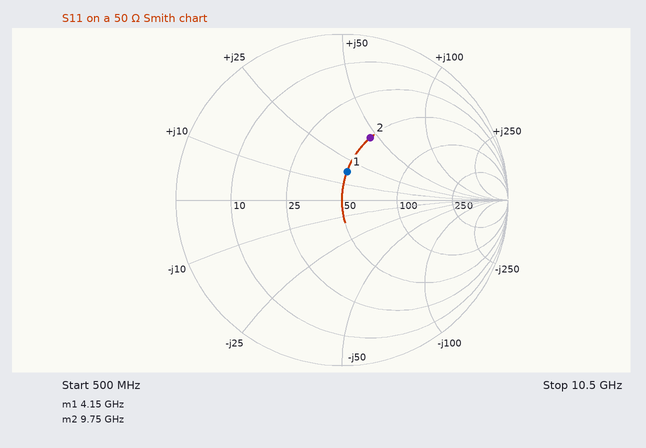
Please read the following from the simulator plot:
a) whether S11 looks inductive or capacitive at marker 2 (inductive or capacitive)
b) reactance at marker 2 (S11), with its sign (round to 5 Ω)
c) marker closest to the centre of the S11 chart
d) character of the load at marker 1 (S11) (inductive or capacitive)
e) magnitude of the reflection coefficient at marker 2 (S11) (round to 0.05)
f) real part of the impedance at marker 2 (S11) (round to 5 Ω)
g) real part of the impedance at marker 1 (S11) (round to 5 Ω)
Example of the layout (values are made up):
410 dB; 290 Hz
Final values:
inductive; +45 Ω; marker 1; inductive; 0.40; 50 Ω; 50 Ω
